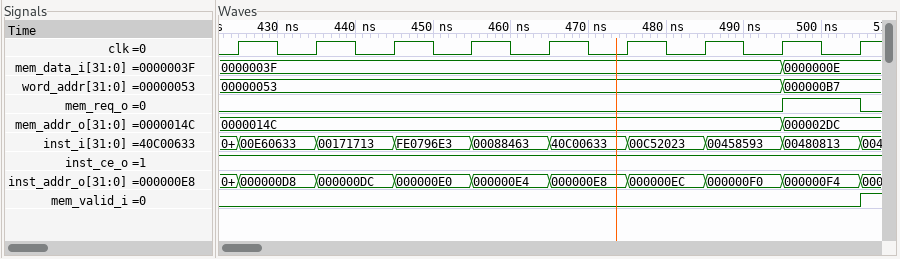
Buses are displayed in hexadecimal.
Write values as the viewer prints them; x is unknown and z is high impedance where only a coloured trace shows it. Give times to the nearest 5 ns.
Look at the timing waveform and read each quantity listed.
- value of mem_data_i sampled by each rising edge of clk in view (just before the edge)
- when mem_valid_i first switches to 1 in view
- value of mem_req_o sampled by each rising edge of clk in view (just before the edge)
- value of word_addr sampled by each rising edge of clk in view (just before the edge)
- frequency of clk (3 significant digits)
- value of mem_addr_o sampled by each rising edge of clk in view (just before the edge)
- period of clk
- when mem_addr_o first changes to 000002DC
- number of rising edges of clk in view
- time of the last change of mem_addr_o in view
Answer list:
0000003F, 0000003F, 0000003F, 0000003F, 0000003F, 0000003F, 0000003F, 0000003F, 0000000E
505 ns
0 0 0 0 0 0 0 0 1
00000053, 00000053, 00000053, 00000053, 00000053, 00000053, 00000053, 00000053, 000000B7
100 MHz
0000014C, 0000014C, 0000014C, 0000014C, 0000014C, 0000014C, 0000014C, 0000014C, 000002DC
10 ns
495 ns
9
495 ns
